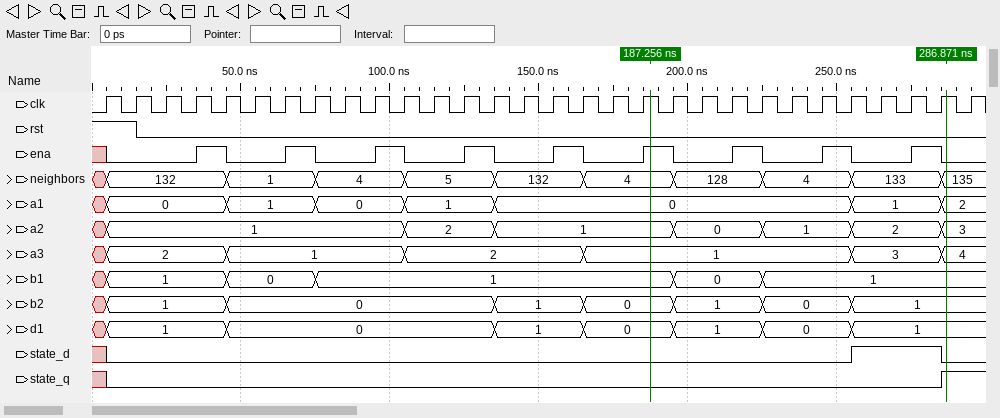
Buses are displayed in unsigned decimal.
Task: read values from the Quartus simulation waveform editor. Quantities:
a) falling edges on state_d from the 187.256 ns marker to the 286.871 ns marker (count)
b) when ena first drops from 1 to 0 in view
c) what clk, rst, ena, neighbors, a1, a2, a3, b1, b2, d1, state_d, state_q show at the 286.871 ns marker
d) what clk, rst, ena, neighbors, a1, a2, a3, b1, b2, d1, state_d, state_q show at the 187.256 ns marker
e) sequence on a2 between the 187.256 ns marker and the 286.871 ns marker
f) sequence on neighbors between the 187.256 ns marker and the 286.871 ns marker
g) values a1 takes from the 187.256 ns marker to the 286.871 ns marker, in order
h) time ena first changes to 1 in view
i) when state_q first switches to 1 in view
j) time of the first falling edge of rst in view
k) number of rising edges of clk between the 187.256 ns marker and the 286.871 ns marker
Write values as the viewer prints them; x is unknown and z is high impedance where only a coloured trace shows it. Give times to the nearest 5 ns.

1
45 ns
clk=1, rst=0, ena=0, neighbors=135, a1=2, a2=3, a3=4, b1=1, b2=1, d1=1, state_d=0, state_q=1
clk=1, rst=0, ena=1, neighbors=4, a1=0, a2=1, a3=1, b1=1, b2=0, d1=0, state_d=0, state_q=0
1, 0, 1, 2, 3
4, 128, 4, 133, 135
0, 1, 2
35 ns
285 ns
15 ns
10
